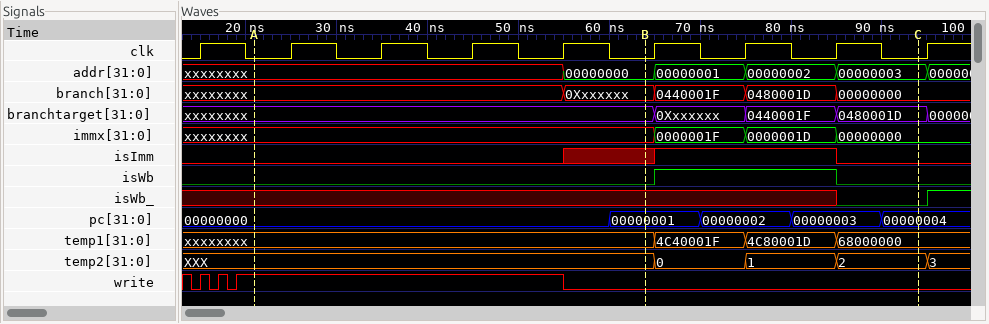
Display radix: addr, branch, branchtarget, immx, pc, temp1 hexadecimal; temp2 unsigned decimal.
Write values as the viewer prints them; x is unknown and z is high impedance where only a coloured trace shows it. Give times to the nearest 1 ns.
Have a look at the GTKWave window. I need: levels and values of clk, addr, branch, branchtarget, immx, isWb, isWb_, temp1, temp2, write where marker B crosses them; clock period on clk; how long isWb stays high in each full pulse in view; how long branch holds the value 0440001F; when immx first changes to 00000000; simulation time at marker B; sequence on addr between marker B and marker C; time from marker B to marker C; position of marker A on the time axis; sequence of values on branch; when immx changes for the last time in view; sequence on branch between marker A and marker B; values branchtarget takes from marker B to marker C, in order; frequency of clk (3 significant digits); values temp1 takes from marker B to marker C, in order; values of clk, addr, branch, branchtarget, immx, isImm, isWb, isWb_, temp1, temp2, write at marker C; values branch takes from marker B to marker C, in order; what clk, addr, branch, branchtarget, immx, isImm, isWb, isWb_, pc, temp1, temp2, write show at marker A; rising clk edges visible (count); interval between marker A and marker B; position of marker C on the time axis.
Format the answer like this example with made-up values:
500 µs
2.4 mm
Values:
clk=0, addr=00000000, branch=0Xxxxxxx, branchtarget=xxxxxxxx, immx=xxxxxxxx, isWb=0, isWb_=x, temp1=xxxxxxxx, temp2=XXX, write=0
10 ns
20 ns
10 ns
85 ns
64 ns
00000000, 00000001, 00000002, 00000003
30 ns
21 ns
xxxxxxxx, 0Xxxxxxx, 0440001F, 0480001D, 00000000
85 ns
xxxxxxxx, 0Xxxxxxx
xxxxxxxx, 0Xxxxxxx, 0440001F, 0480001D
100 MHz
xxxxxxxx, 4C40001F, 4C80001D, 68000000
clk=0, addr=00000003, branch=00000000, branchtarget=0480001D, immx=00000000, isImm=0, isWb=0, isWb_=0, temp1=68000000, temp2=2, write=0
0Xxxxxxx, 0440001F, 0480001D, 00000000
clk=0, addr=xxxxxxxx, branch=xxxxxxxx, branchtarget=xxxxxxxx, immx=xxxxxxxx, isImm=0, isWb=0, isWb_=x, pc=00000000, temp1=xxxxxxxx, temp2=XXX, write=1
9
43 ns
94 ns
